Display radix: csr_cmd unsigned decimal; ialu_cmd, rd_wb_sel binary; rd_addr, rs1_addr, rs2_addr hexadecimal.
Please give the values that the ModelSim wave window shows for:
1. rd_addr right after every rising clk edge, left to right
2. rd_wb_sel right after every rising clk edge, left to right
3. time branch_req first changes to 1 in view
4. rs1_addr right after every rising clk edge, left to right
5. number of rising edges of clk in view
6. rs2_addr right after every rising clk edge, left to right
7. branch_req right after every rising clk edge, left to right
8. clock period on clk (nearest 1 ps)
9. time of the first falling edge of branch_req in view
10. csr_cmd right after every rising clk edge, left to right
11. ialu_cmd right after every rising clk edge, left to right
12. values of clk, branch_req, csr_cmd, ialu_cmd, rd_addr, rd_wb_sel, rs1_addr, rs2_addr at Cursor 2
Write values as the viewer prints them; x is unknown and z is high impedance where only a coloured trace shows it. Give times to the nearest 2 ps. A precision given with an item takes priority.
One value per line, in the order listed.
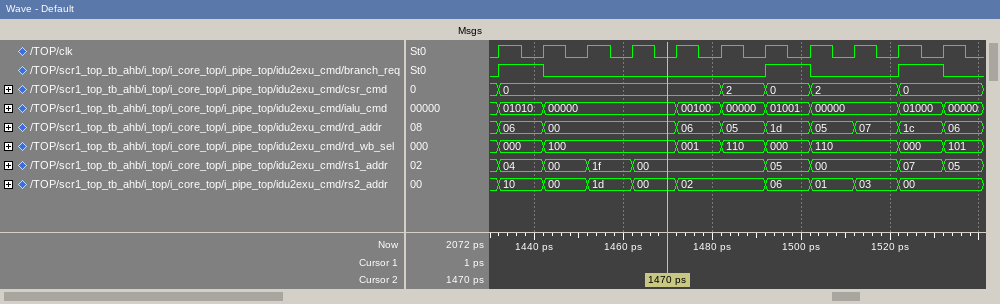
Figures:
06, 00, 00, 00, 06, 05, 1d, 05, 07, 1c, 06
000, 100, 100, 100, 001, 110, 000, 110, 110, 000, 101
1432 ps
04, 00, 1f, 00, 00, 00, 05, 00, 00, 07, 05
11
10, 00, 1d, 00, 02, 02, 06, 01, 03, 00, 00
1 0 0 0 0 0 1 0 0 1 0
10 ps
1442 ps
0, 0, 0, 0, 0, 2, 0, 2, 2, 0, 0
01010, 00000, 00000, 00000, 00100, 00000, 01001, 00000, 00000, 01000, 00000
clk=0, branch_req=0, csr_cmd=0, ialu_cmd=00000, rd_addr=00, rd_wb_sel=100, rs1_addr=00, rs2_addr=00
